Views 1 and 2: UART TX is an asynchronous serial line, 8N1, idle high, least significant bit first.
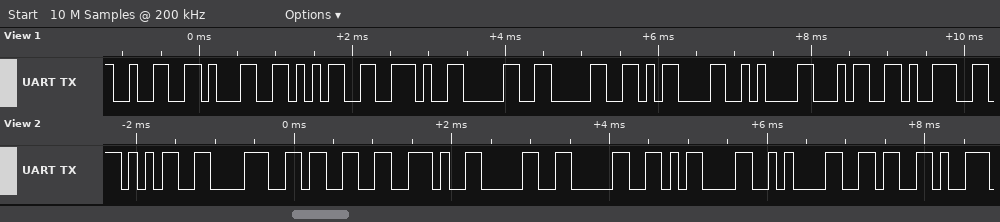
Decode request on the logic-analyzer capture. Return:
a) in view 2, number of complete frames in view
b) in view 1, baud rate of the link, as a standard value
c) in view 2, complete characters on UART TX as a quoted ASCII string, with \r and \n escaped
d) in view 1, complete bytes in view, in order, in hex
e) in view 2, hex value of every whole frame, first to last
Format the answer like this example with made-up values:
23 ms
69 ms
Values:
9
9600 baud
"583.00\r\n6"
0x32 0x31 0x35 0x2E 0x30 0x30 0x0D 0x0A 0x34 0x39
35 38 33 2E 30 30 0D 0A 36
